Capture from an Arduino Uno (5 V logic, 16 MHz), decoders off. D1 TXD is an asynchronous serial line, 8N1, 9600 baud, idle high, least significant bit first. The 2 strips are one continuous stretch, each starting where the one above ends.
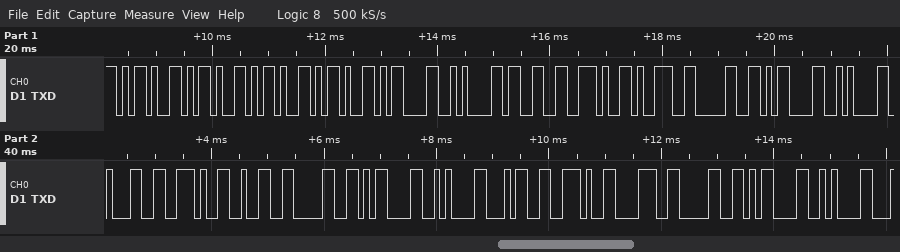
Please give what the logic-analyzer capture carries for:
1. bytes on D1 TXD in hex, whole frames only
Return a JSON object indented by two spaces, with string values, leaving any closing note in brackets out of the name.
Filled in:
{
  "bytes on D1 TXD in hex, whole frames only": "0x2D 0x2D 0x2D 0x2D 0x0D 0x0A 0x33 0x2E 0x39 0x30 0x0D 0x0A 0x31 0x2E 0x32 0x30 0x0D 0x0A 0x34 0x2E 0x38 0x30 0x0D 0x0A"
}
